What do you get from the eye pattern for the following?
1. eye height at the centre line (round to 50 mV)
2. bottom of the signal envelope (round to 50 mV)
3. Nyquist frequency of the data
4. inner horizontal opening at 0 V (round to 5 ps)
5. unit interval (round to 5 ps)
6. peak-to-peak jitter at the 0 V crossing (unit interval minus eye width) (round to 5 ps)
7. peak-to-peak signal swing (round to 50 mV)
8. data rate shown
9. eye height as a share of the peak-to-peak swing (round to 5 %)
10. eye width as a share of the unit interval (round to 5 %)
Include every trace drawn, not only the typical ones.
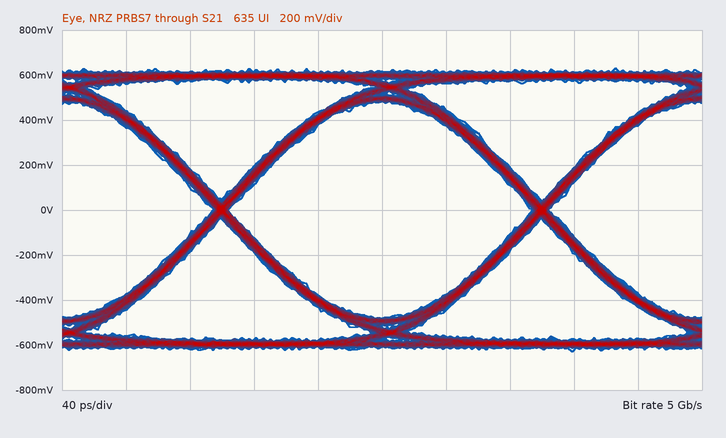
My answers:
950 mV
-650 mV
2.5 GHz
190 ps
200 ps
10 ps
1.25 V
5 Gb/s
75 %
95 %
